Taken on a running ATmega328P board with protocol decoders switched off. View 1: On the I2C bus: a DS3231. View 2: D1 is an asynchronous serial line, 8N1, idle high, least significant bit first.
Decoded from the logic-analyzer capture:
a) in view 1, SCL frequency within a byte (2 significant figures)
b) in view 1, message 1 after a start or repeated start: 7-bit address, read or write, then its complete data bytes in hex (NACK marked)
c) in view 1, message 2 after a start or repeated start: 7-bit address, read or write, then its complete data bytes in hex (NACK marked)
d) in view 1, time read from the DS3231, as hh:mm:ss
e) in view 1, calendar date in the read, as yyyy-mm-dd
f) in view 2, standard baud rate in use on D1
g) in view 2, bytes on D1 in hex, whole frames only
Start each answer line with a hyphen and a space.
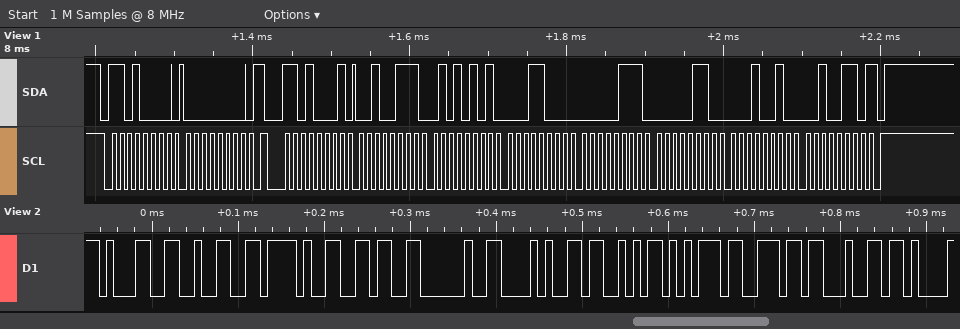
- 100 kHz
- 0x68 write: 00
- 0x68 read: 27 55 18 07 06 12 26 NACK
- 18:55:27
- 2026-12-06
- 115200 baud
- 31 32 2F 36 20 28 53 75 6E 64
